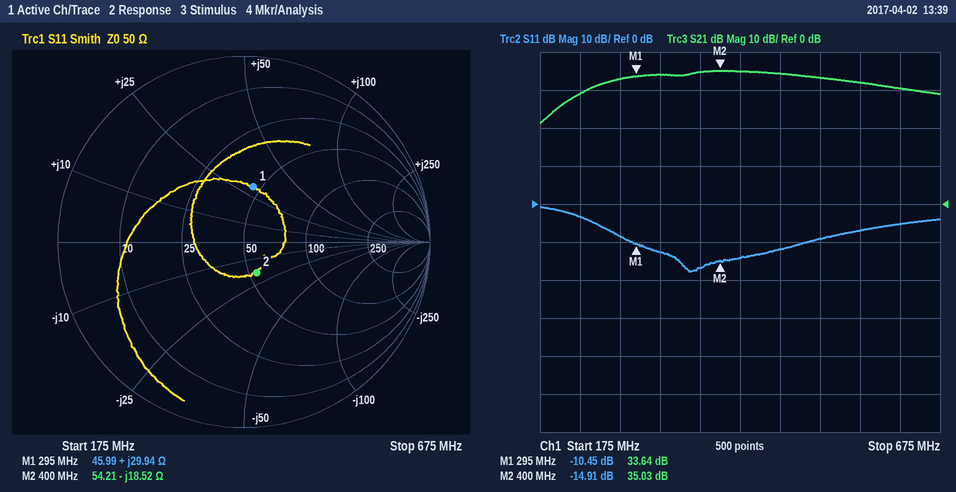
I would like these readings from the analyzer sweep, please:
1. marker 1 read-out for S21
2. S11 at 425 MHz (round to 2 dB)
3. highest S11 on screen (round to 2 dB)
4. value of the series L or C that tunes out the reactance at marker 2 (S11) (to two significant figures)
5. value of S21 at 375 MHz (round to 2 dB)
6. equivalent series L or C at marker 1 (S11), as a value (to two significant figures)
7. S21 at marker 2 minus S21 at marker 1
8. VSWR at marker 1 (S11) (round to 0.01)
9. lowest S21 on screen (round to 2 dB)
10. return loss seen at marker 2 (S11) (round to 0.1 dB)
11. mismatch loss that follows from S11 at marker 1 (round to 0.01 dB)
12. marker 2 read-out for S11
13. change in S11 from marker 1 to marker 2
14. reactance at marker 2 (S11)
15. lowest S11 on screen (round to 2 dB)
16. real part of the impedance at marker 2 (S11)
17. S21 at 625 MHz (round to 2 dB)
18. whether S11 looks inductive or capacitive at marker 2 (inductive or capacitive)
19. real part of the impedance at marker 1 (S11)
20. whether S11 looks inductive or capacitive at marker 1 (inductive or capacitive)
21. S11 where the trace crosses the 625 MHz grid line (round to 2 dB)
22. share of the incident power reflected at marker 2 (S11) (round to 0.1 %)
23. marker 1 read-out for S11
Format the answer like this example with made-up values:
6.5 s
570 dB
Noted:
33.64 dB
-14 dB
0 dB
7.4 nH
34 dB
16 nH
1.39 dB
1.86
22 dB
14.9 dB
0.41 dB
-14.91 dB
-4.46 dB
-18.52 Ω
-18 dB
54.21 Ω
30 dB
capacitive
45.99 Ω
inductive
-6 dB
3.2 %
-10.45 dB
